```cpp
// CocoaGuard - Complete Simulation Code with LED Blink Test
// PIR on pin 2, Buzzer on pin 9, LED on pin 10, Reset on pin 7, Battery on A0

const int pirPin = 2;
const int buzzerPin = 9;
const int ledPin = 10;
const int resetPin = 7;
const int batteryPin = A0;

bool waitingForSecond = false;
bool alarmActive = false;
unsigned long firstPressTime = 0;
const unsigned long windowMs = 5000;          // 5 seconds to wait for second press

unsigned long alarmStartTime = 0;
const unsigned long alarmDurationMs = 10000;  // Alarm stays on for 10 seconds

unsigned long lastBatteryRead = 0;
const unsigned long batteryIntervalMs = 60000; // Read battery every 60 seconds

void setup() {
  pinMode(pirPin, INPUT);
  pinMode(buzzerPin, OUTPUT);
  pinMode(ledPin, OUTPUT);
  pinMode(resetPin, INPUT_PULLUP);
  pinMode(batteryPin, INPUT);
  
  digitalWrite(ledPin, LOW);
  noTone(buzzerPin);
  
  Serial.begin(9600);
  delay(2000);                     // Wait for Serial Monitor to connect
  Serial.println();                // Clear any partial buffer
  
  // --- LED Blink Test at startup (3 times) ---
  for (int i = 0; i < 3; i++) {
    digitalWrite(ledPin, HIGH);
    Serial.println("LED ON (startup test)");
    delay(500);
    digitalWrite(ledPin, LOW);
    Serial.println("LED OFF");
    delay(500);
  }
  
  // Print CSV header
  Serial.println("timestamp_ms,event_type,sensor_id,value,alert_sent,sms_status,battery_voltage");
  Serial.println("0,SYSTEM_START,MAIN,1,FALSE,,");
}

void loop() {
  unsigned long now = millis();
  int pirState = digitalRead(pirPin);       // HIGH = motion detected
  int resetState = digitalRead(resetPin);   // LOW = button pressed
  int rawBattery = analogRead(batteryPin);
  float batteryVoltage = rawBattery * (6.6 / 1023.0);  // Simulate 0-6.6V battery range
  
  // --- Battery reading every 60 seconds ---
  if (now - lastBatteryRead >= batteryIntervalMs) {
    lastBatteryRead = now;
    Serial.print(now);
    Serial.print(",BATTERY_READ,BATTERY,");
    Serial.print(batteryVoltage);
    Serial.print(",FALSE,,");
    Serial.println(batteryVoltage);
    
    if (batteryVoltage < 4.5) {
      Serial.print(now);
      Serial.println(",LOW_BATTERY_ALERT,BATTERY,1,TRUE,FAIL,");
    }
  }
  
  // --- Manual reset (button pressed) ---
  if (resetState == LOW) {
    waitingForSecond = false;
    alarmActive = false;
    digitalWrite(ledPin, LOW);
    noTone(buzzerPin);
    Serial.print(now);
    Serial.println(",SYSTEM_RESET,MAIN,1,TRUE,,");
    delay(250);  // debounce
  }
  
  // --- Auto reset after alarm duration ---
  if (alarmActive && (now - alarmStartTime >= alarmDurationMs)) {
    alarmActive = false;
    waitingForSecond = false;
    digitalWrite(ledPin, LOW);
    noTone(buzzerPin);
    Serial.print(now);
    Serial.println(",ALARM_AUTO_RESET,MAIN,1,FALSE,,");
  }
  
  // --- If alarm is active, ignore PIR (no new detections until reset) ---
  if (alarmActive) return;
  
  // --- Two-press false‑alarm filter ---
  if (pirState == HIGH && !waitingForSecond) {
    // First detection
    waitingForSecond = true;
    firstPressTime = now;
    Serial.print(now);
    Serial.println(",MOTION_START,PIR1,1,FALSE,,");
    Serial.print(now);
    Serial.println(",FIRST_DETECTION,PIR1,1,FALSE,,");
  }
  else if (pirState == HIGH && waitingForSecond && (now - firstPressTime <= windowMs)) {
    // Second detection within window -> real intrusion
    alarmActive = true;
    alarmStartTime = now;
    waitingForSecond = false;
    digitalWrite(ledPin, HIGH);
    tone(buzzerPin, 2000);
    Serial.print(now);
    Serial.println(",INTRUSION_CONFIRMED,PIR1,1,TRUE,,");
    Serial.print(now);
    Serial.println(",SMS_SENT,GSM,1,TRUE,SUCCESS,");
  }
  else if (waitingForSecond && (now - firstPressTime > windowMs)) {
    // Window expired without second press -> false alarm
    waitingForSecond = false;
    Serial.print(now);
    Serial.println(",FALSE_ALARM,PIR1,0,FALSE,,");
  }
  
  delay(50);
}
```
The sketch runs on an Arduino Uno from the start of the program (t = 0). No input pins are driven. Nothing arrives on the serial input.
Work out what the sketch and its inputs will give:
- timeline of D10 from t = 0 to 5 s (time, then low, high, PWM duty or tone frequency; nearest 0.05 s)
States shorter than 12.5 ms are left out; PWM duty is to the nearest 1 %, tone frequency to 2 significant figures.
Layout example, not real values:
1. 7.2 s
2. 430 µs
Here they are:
1. 0 s low; 2 s high; 2.5 s low; 3 s high; 3.5 s low; 4 s high; 4.5 s low
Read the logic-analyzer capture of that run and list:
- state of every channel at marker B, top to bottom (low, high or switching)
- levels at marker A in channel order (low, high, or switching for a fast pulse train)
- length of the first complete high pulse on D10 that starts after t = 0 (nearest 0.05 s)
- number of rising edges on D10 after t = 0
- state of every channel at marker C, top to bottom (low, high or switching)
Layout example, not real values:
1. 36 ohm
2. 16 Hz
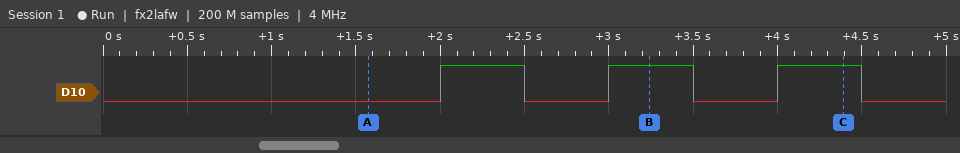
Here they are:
1. D10 high
2. D10 low
3. 0.50 s
4. 3
5. D10 high
